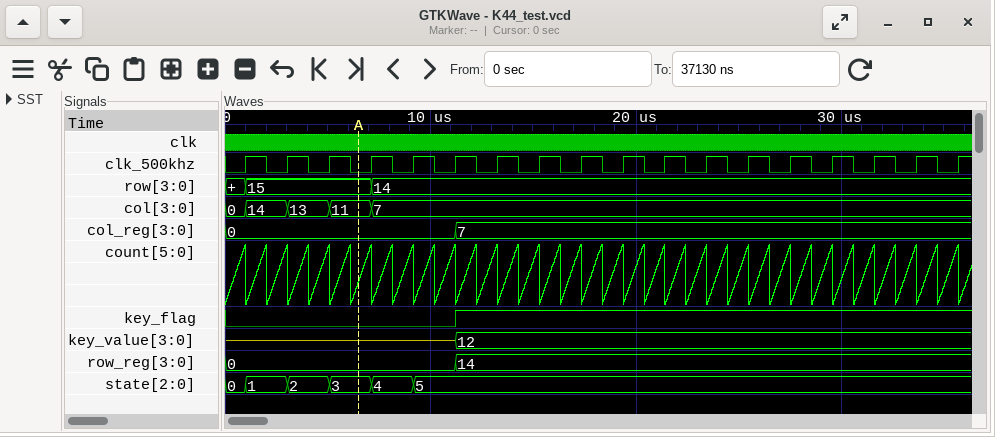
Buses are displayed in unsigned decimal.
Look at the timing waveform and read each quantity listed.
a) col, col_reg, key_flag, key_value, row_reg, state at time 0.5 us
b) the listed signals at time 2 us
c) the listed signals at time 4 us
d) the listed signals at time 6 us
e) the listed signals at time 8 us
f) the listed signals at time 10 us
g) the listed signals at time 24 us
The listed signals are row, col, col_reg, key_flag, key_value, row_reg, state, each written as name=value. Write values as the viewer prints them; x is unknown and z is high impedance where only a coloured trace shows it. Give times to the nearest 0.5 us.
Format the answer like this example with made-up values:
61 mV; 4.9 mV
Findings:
col=0, col_reg=0, key_flag=0, key_value=z, row_reg=0, state=0; row=15, col=14, col_reg=0, key_flag=0, key_value=z, row_reg=0, state=1; row=15, col=13, col_reg=0, key_flag=0, key_value=z, row_reg=0, state=2; row=15, col=11, col_reg=0, key_flag=0, key_value=z, row_reg=0, state=3; row=14, col=7, col_reg=0, key_flag=0, key_value=z, row_reg=0, state=4; row=14, col=7, col_reg=0, key_flag=0, key_value=z, row_reg=0, state=5; row=14, col=7, col_reg=7, key_flag=1, key_value=12, row_reg=14, state=5
